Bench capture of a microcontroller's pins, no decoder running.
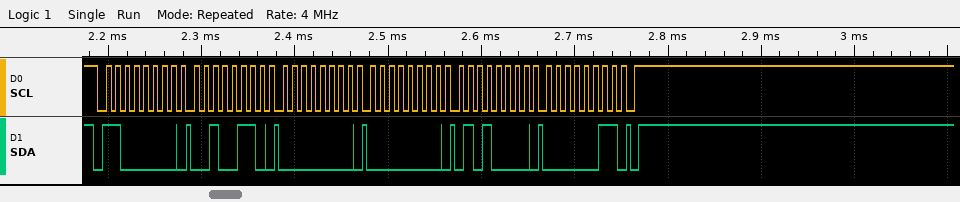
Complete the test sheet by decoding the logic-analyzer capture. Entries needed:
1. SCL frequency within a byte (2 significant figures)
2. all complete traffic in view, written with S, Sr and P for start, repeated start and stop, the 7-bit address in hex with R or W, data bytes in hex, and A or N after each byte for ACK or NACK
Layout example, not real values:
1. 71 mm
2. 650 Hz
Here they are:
1. 100 kHz
2. S 60W A 26 A 00 A 00 A 50 A 03 A P
